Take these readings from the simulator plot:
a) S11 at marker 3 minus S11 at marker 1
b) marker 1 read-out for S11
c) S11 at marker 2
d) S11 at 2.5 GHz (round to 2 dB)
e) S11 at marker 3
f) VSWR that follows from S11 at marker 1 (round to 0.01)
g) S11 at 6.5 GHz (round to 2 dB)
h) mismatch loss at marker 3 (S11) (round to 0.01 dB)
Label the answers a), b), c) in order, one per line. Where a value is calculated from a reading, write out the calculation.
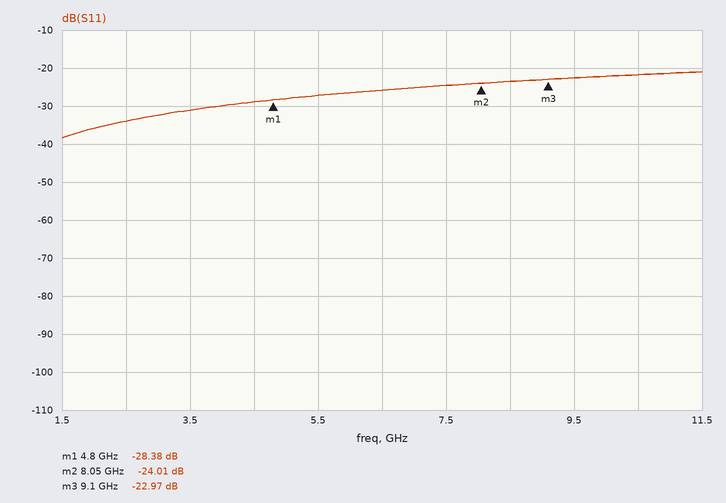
a) -22.97 − (-28.38) = 5.41 dB
b) -28.38 dB
c) -24.01 dB
d) -34 dB
e) -22.97 dB
f) (1 + 0.0381)/(1 − 0.0381) ≈ 1.08
g) -26 dB
h) −10 log10(1 − 10^(-22.97/10)) ≈ 0.02 dB
